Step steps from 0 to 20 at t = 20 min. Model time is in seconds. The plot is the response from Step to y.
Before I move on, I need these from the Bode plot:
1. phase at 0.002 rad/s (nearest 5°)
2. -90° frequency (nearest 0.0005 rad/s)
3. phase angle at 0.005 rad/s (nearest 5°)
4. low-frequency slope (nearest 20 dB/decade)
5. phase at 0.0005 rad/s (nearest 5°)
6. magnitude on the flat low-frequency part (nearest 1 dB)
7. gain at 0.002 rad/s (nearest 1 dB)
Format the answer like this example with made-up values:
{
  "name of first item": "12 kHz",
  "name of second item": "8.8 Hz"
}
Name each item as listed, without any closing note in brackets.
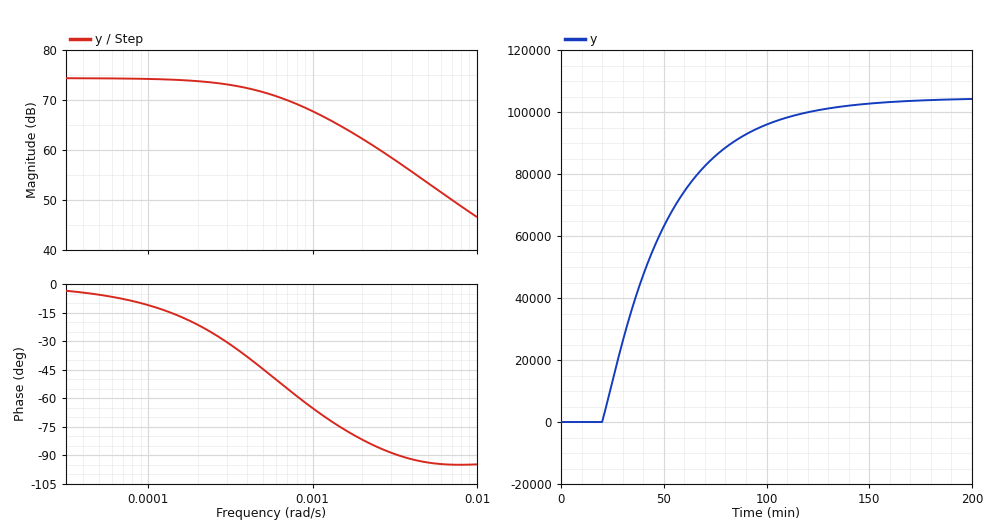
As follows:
{
  "phase at 0.002 rad/s": "-80°",
  "-90° frequency": "0.0035 rad/s",
  "phase angle at 0.005 rad/s": "-95°",
  "low-frequency slope": "0 dB/decade",
  "phase at 0.0005 rad/s": "-45°",
  "magnitude on the flat low-frequency part": "74 dB",
  "gain at 0.002 rad/s": "62 dB"
}
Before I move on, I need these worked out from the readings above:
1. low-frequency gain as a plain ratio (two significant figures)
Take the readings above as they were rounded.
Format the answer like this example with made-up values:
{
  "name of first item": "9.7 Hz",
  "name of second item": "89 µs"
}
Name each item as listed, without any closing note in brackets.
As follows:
{
  "low-frequency gain as a plain ratio": "5000"
}
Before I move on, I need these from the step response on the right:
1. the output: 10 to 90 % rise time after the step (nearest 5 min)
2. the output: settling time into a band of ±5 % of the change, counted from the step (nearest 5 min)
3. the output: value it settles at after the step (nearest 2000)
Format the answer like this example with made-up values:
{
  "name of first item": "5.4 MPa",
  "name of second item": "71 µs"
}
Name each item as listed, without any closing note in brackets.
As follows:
{
  "the output: 10 to 90 % rise time after the step": "70 min",
  "the output: settling time into a band of ±5 % of the change, counted from the step": "95 min",
  "the output: value it settles at after the step": "104000"
}
